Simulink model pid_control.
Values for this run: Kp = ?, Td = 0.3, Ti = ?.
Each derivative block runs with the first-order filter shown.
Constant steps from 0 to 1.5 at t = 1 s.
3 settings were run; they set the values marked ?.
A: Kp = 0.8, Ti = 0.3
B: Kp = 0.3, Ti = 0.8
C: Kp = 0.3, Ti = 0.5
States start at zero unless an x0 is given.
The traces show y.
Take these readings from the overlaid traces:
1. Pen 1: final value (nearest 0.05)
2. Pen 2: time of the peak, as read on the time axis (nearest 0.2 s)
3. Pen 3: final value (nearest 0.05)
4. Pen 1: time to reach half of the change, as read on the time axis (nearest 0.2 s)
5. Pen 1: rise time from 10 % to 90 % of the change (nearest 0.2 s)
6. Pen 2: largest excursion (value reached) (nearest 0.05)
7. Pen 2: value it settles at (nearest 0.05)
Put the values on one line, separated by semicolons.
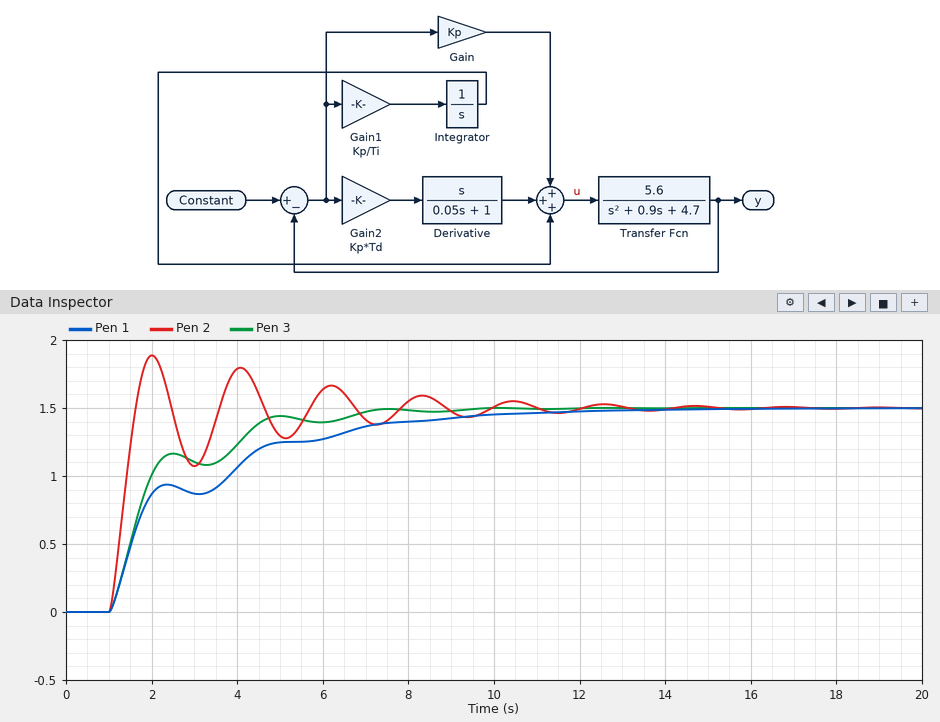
1.50; 2.0 s; 1.50; 1.8 s; 5.6 s; 1.90; 1.50
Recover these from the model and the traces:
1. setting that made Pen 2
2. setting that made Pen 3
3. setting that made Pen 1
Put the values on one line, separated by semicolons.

A; C; B
